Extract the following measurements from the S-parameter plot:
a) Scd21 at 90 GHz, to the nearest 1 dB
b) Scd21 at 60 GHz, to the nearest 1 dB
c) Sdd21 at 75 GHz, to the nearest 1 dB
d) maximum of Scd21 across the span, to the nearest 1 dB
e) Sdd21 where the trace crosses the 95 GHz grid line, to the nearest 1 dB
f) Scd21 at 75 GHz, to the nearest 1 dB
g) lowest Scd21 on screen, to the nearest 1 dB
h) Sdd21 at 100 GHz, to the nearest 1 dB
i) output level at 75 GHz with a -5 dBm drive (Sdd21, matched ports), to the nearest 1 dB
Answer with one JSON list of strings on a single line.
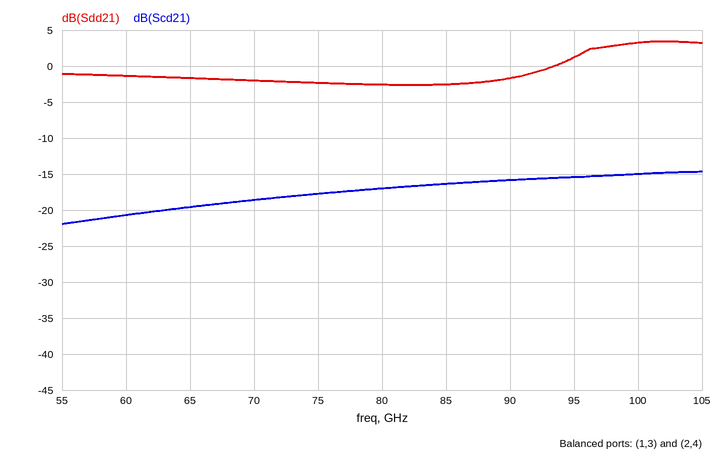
["-16 dB", "-21 dB", "-2 dB", "-15 dB", "1 dB", "-18 dB", "-22 dB", "3 dB", "-7 dBm"]
